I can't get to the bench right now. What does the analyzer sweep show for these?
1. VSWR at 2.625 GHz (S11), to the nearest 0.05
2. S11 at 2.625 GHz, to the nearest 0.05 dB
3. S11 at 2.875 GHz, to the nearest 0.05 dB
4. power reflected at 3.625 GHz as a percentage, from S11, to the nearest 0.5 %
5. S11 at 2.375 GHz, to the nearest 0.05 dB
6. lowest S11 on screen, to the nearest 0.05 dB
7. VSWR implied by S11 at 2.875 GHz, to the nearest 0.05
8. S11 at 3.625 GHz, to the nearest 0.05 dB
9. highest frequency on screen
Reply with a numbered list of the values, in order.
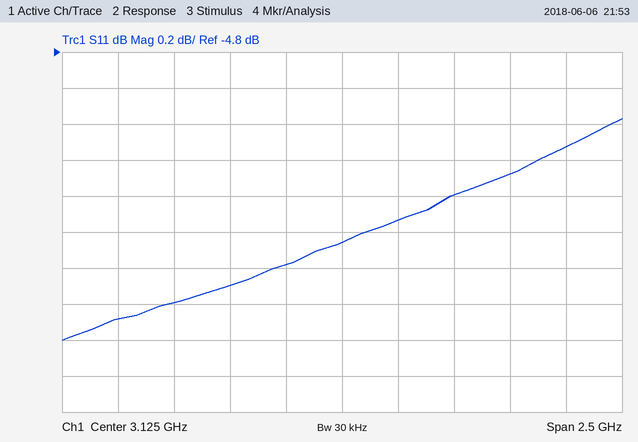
1. 2.95
2. -6.10 dB
3. -6.00 dB
4. 27.5 %
5. -6.20 dB
6. -6.40 dB
7. 3.00
8. -5.60 dB
9. 4.375 GHz
